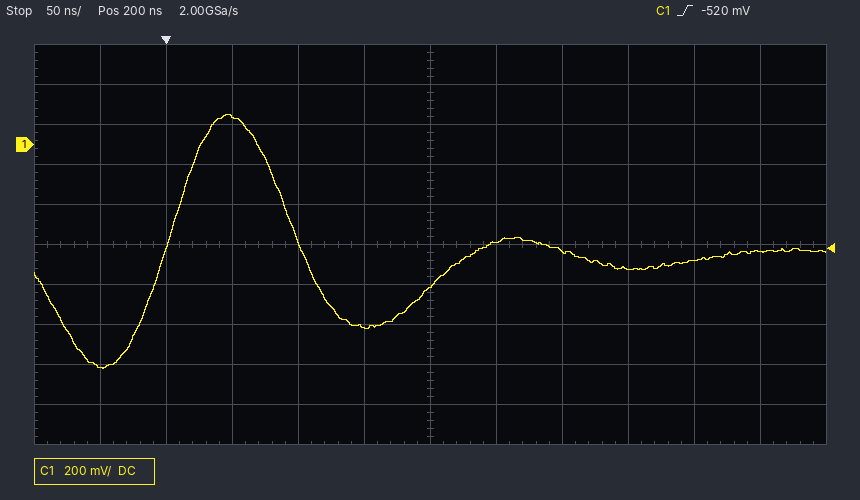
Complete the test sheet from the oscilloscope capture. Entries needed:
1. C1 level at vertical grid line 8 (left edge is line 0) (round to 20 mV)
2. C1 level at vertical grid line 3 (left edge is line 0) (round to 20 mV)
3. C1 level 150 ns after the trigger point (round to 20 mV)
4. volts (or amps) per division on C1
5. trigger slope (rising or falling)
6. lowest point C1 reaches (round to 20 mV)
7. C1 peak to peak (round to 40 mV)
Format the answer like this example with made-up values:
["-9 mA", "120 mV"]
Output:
["-540 mV", "140 mV", "-920 mV", "200 mV", "rising", "-1.12 V", "1.28 V"]
